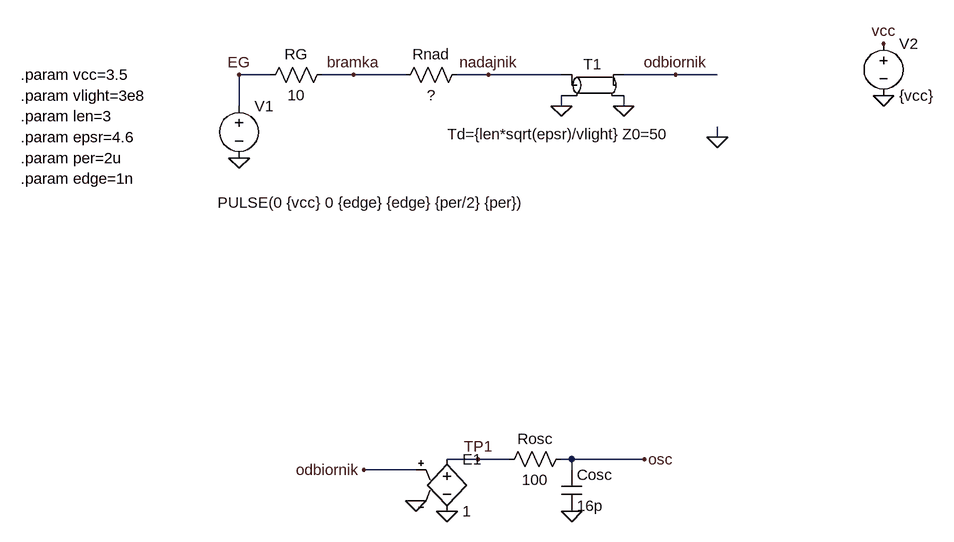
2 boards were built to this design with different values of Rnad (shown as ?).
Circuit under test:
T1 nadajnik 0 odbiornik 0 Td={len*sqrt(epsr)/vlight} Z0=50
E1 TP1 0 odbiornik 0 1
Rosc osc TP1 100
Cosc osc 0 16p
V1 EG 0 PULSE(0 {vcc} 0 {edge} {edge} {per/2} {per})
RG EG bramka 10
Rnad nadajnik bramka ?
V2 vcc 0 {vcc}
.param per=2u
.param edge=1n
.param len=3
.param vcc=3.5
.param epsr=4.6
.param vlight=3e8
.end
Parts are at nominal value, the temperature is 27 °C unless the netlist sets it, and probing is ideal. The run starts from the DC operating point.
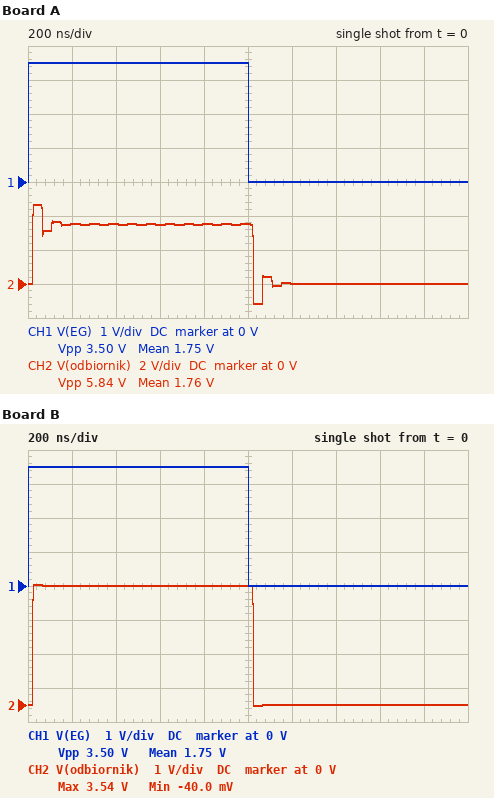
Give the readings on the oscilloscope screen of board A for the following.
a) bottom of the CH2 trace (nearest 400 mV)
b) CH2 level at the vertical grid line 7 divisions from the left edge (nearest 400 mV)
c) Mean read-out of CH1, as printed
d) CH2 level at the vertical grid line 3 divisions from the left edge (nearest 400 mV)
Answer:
-1.2 V
0 V
1.75 V
3.6 V
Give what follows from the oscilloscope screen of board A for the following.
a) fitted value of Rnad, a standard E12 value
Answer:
15 Ω
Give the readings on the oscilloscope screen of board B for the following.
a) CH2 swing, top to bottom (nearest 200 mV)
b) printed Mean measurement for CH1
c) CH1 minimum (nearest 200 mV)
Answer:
3.6 V
1.75 V
0 V
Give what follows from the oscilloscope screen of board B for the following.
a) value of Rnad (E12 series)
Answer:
39 Ω
